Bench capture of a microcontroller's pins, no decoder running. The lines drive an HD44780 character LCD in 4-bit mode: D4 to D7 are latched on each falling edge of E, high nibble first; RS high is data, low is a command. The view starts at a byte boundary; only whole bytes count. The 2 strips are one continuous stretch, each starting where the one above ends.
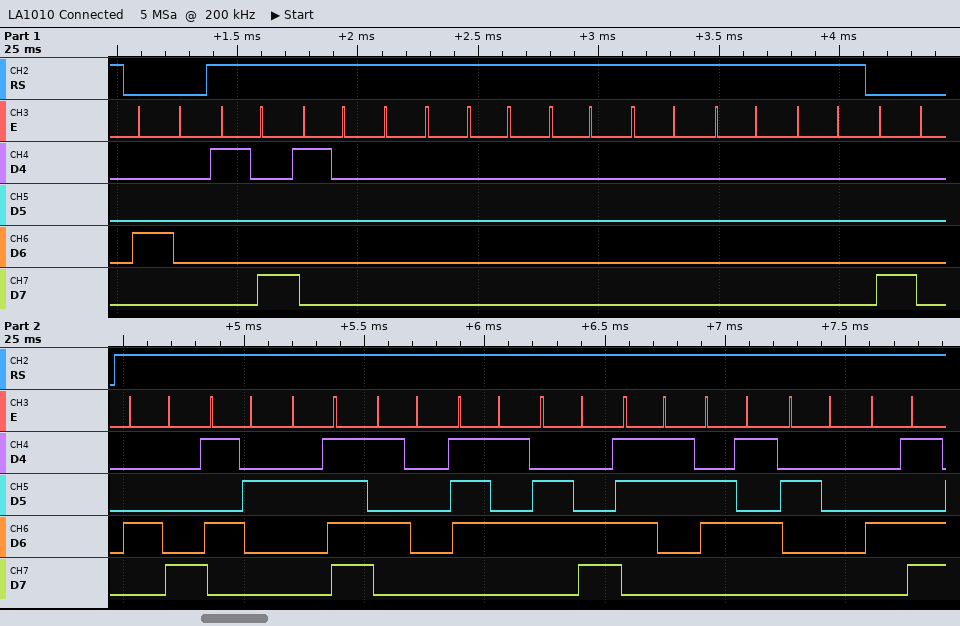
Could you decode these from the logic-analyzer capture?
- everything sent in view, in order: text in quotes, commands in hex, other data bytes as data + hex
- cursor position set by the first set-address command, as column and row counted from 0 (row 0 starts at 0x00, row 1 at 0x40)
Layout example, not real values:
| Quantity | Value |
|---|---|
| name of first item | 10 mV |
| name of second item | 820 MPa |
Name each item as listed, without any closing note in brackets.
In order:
| Quantity | Value |
|---|---|
| everything sent in view, in order: text in quotes, commands in hex, other data bytes as data + hex | 0x40 data 18 10 00 00 00 00 00 00 0x80 "HR/Pulse M" |
| cursor position set by the first set-address command, as column and row counted from 0 | column 0, row 0 |
